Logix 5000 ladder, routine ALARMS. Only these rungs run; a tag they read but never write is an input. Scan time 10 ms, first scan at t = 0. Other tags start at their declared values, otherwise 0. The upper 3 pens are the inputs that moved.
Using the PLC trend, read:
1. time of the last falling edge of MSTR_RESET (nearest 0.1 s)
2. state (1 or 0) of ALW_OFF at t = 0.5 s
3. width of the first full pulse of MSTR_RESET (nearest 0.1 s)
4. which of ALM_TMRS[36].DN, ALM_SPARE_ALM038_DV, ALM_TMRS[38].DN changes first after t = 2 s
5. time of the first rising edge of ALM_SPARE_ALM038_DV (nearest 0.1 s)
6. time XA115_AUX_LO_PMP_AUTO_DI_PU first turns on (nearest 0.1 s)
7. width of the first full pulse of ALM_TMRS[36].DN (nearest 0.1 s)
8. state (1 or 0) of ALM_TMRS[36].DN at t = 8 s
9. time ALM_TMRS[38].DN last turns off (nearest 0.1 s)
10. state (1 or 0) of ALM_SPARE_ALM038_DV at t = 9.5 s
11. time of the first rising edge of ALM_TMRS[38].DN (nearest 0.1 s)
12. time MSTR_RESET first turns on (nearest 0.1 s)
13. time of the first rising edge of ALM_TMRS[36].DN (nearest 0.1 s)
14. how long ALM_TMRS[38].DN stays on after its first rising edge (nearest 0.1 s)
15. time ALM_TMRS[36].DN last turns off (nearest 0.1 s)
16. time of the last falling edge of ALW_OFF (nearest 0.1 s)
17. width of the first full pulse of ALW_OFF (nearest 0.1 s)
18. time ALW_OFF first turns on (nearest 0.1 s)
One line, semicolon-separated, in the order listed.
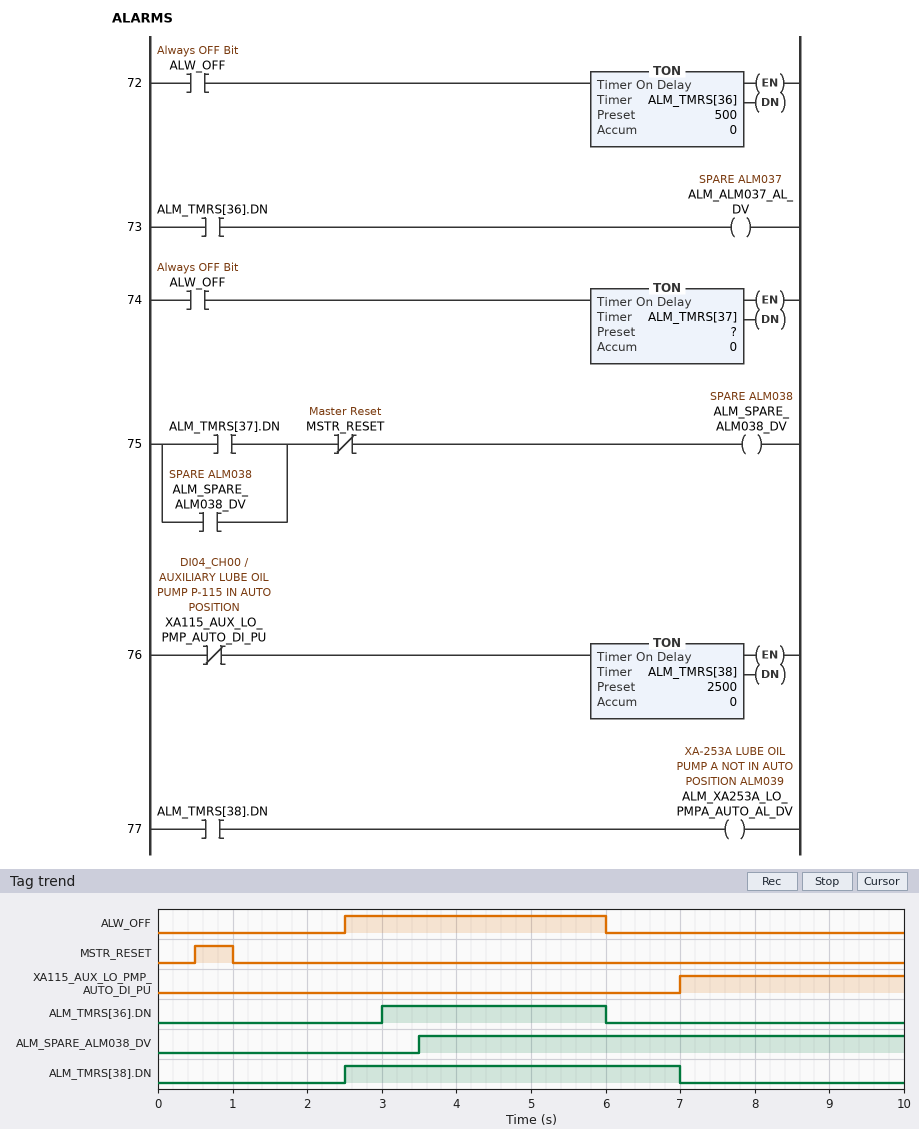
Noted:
1.0 s; 0; 0.5 s; ALM_TMRS[38].DN; 3.5 s; 7.0 s; 3.0 s; 0; 7.0 s; 1; 2.5 s; 0.5 s; 3.0 s; 4.5 s; 6.0 s; 6.0 s; 3.5 s; 2.5 s
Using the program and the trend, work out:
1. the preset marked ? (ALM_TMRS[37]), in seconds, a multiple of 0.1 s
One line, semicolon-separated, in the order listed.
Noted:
1.0 s
